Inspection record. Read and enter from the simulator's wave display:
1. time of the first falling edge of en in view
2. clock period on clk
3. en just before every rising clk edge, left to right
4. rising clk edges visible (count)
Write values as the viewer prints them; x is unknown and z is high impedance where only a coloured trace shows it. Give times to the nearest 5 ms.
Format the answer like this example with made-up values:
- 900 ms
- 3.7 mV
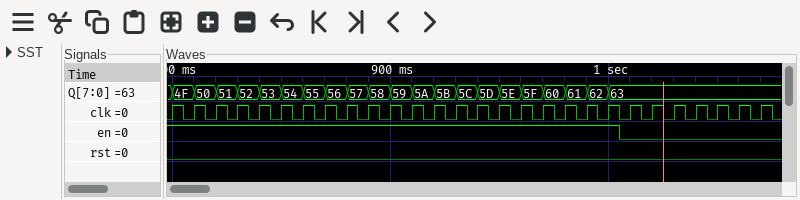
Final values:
- 1005 ms
- 10 ms
- 1 1 1 1 1 1 1 1 1 1 1 1 1 1 1 1 1 1 1 1 1 0 0 0 0 0 0 0
- 28
